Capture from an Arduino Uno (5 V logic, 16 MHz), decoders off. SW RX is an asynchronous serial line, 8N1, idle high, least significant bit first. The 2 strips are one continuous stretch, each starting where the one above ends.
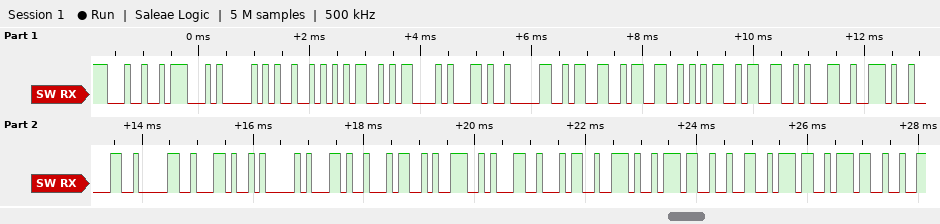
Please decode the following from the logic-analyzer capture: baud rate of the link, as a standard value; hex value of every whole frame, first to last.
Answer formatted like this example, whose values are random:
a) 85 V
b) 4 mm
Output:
a) 9600 baud
b) 24 47 50 52 4D 43 2C 30 33 33 35 33 31 2E 30 30 2C 41 2C 34 39 31 34 2E 37 32 37 37
